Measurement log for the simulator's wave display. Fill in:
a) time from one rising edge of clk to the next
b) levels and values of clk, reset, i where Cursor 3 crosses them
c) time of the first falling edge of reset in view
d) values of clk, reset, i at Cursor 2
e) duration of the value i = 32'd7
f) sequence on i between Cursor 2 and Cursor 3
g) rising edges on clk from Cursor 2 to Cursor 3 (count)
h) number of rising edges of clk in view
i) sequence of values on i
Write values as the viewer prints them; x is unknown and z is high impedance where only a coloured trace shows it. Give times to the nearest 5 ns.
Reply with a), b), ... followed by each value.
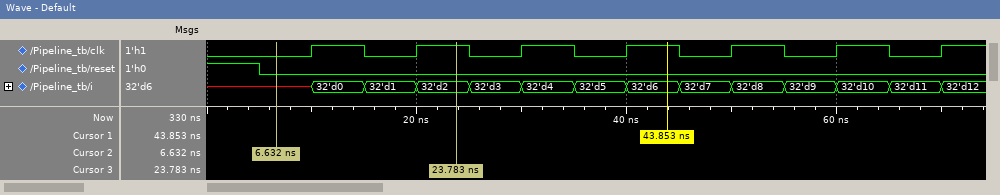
a) 10 ns
b) clk=1, reset=0, i=32'd2
c) 5 ns
d) clk=0, reset=0, i=x
e) 5 ns
f) x, 32'd0, 32'd1, 32'd2
g) 2
h) 7
i) x, 32'd0, 32'd1, 32'd2, 32'd3, 32'd4, 32'd5, 32'd6, 32'd7, 32'd8, 32'd9, 32'd10, 32'd11, 32'd12
